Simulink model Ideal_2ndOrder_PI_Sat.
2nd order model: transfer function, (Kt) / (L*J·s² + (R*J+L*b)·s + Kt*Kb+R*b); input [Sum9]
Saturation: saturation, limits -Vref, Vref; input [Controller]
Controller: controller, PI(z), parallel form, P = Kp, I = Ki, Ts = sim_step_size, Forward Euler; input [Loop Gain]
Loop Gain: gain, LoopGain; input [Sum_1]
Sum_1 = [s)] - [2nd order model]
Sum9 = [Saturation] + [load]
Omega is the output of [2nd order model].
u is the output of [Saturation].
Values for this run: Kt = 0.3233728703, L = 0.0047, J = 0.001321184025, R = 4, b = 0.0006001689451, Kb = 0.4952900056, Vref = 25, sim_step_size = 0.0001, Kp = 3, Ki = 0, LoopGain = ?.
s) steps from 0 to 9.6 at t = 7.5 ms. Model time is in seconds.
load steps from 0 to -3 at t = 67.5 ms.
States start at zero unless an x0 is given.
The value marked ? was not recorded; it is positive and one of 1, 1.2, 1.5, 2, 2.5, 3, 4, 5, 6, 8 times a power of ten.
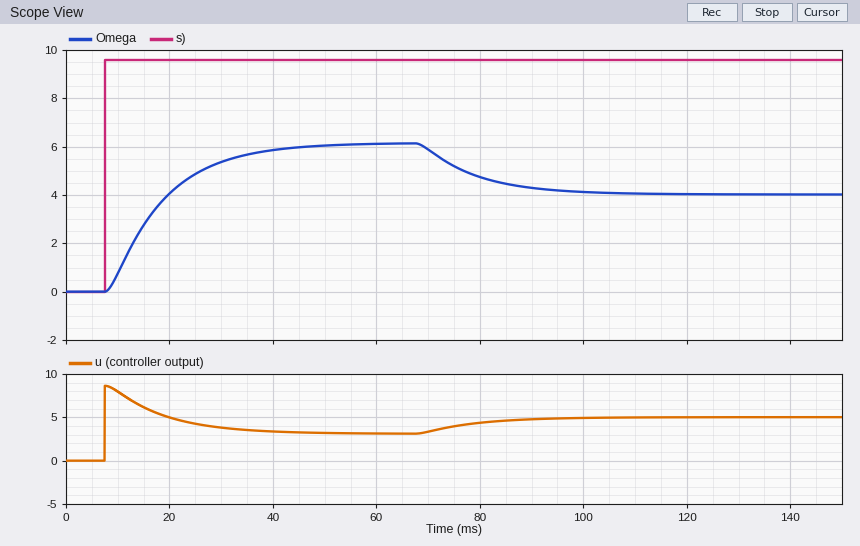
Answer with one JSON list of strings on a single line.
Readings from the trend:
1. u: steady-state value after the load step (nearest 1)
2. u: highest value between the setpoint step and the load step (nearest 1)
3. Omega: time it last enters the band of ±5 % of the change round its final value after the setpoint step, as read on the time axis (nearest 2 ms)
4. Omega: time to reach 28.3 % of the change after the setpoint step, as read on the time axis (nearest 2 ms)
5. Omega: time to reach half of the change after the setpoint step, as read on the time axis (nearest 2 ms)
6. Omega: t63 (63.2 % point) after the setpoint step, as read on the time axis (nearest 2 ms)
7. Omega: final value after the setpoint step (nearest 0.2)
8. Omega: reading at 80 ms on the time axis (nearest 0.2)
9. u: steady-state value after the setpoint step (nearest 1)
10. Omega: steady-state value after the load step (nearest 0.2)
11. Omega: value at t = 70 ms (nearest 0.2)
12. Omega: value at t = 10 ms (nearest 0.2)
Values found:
["5", "9", "40 ms", "12 ms", "16 ms", "20 ms", "6.2", "4.8", "3", "4.0", "5.8", "0.8"]
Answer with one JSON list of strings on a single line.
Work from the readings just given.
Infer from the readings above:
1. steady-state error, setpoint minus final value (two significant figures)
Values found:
["3.4"]
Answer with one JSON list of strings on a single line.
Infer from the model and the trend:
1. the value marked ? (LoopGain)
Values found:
["0.3"]
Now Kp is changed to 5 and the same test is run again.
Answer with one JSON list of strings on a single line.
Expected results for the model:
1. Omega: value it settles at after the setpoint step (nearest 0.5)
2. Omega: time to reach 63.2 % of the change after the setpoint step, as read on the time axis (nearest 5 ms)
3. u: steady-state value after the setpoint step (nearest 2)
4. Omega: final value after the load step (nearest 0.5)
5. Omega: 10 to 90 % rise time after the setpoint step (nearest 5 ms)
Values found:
["7.0", "15 ms", "4", "5.5", "15 ms"]
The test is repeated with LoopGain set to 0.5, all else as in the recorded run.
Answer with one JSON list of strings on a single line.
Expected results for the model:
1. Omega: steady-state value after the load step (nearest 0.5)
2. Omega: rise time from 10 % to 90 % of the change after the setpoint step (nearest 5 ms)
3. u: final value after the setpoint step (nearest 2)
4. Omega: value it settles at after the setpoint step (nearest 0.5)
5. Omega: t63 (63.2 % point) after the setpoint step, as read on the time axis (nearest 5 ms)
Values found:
["5.5", "15 ms", "4", "7.0", "15 ms"]
